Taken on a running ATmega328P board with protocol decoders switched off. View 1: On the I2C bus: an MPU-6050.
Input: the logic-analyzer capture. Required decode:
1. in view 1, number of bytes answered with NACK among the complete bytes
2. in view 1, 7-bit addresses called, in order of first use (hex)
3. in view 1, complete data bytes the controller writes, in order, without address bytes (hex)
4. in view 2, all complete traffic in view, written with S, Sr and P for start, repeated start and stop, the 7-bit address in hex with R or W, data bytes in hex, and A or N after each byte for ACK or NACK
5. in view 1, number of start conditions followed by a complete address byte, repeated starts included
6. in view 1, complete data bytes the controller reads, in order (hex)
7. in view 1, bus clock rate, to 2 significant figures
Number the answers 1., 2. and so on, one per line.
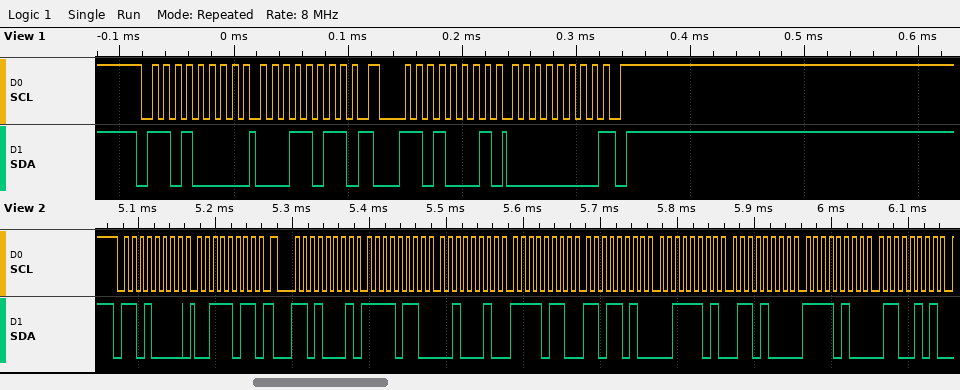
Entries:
1. 1
2. 0x68
3. 1B
4. S 68W A 3B A Sr 68R A F6 A 22 A F6 A DA A 3D A 68 A F4 A 65 A
5. 2
6. 00
7. 100 kHz
